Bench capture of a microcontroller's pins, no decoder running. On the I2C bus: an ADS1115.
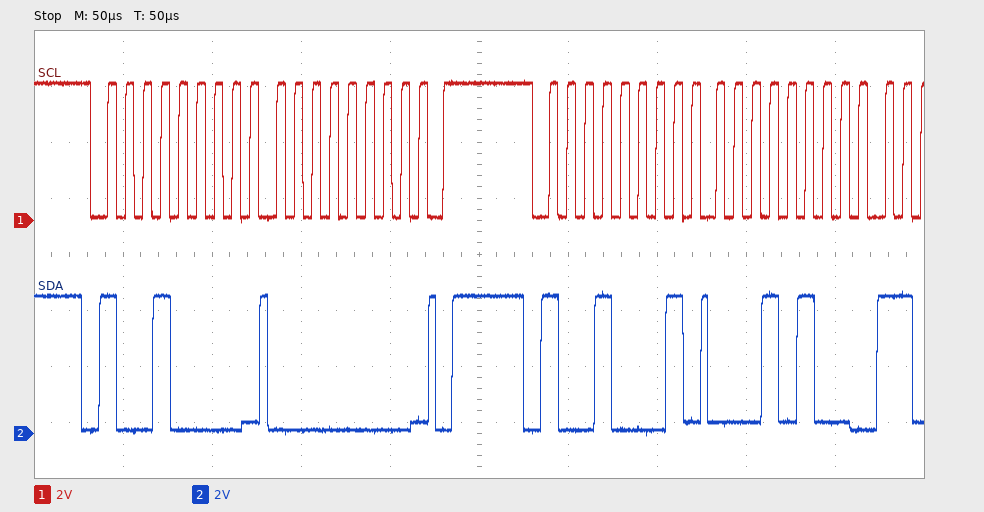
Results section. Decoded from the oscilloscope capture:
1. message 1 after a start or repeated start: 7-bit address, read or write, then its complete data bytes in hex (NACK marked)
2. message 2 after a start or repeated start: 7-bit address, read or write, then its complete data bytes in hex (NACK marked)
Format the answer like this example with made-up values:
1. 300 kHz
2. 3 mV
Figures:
1. 0x48 write: 00
2. 0x48 read: 14
